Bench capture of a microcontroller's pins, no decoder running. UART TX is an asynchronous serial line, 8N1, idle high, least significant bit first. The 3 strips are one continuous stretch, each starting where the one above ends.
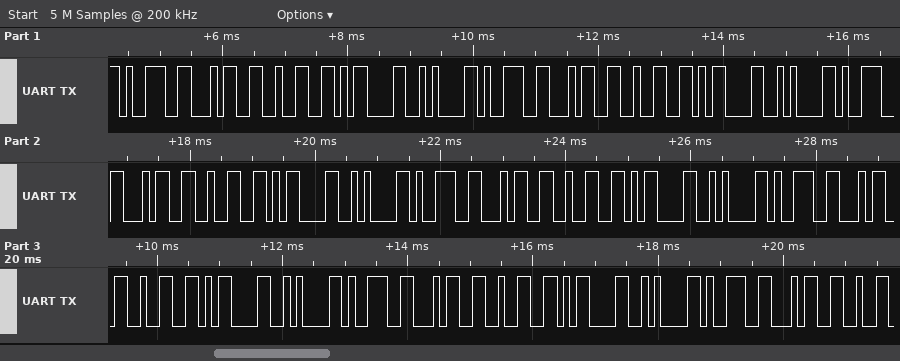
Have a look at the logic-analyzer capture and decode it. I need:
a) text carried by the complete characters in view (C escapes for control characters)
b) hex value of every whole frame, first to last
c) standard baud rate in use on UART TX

"942\r\n942\r\n942\r\n942\r\n942\r\n942\r\n94"
39 34 32 0D 0A 39 34 32 0D 0A 39 34 32 0D 0A 39 34 32 0D 0A 39 34 32 0D 0A 39 34 32 0D 0A 39 34
9600 baud
